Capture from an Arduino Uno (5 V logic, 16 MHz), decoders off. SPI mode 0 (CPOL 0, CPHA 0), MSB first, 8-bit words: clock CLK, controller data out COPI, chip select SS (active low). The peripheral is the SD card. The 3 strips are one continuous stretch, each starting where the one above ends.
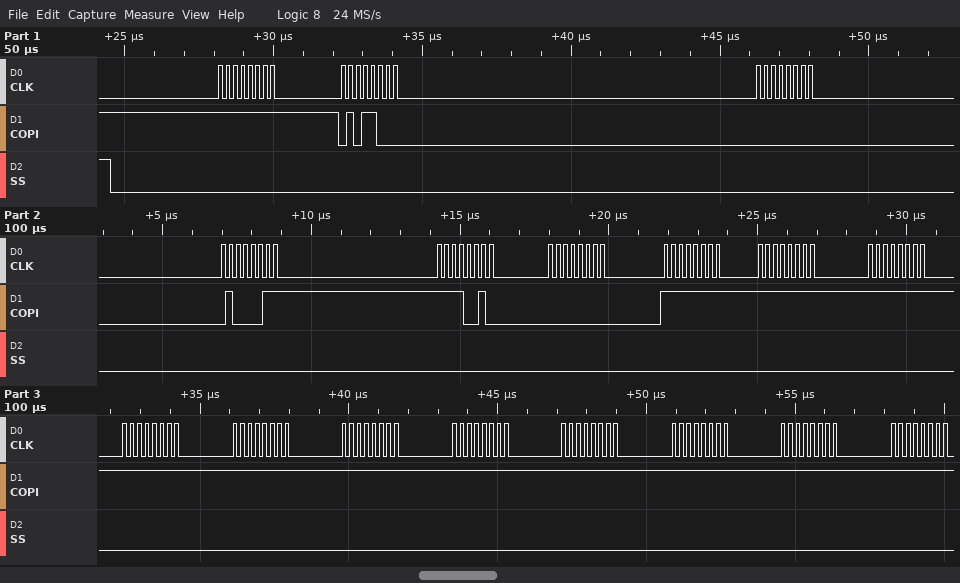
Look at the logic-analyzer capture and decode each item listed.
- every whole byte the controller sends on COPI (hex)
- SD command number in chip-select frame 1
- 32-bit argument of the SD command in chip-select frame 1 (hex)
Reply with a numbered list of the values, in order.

1. FF 58 00 43 F2 00 FF FF FF FF FF FF FF FF FF FF FF
2. CMD24
3. 0x0043F200
